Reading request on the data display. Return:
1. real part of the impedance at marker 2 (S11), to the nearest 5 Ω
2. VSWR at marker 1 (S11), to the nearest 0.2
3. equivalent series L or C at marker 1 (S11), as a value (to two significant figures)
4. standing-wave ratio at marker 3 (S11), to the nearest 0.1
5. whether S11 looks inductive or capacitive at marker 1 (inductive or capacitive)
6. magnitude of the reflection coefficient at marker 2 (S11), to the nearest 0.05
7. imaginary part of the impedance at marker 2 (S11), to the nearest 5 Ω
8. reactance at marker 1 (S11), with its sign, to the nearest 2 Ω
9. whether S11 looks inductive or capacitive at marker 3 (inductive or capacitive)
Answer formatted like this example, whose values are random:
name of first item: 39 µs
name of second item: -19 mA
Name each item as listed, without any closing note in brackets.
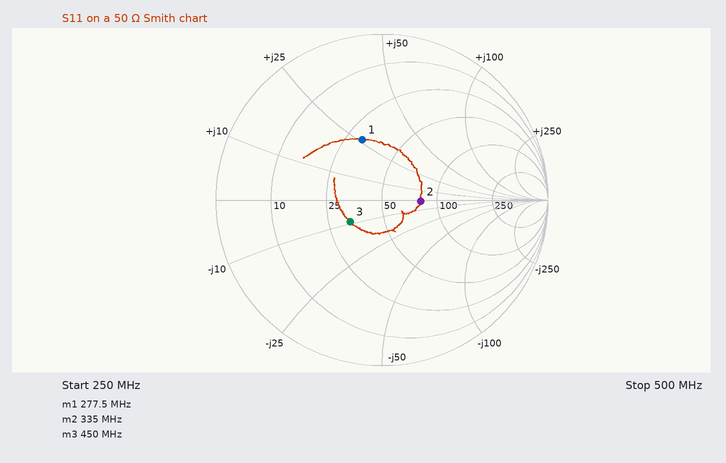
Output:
real part of the impedance at marker 2 (S11), to the nearest 5 Ω: 80 Ω
VSWR at marker 1 (S11), to the nearest 0.2: 2.2
equivalent series L or C at marker 1 (S11), as a value: 15 nH
standing-wave ratio at marker 3 (S11), to the nearest 0.1: 1.6
whether S11 looks inductive or capacitive at marker 1: inductive
magnitude of the reflection coefficient at marker 2 (S11), to the nearest 0.05: 0.25
imaginary part of the impedance at marker 2 (S11), to the nearest 5 Ω: 0 Ω
reactance at marker 1 (S11), with its sign, to the nearest 2 Ω: +26 Ω
whether S11 looks inductive or capacitive at marker 3: capacitive
